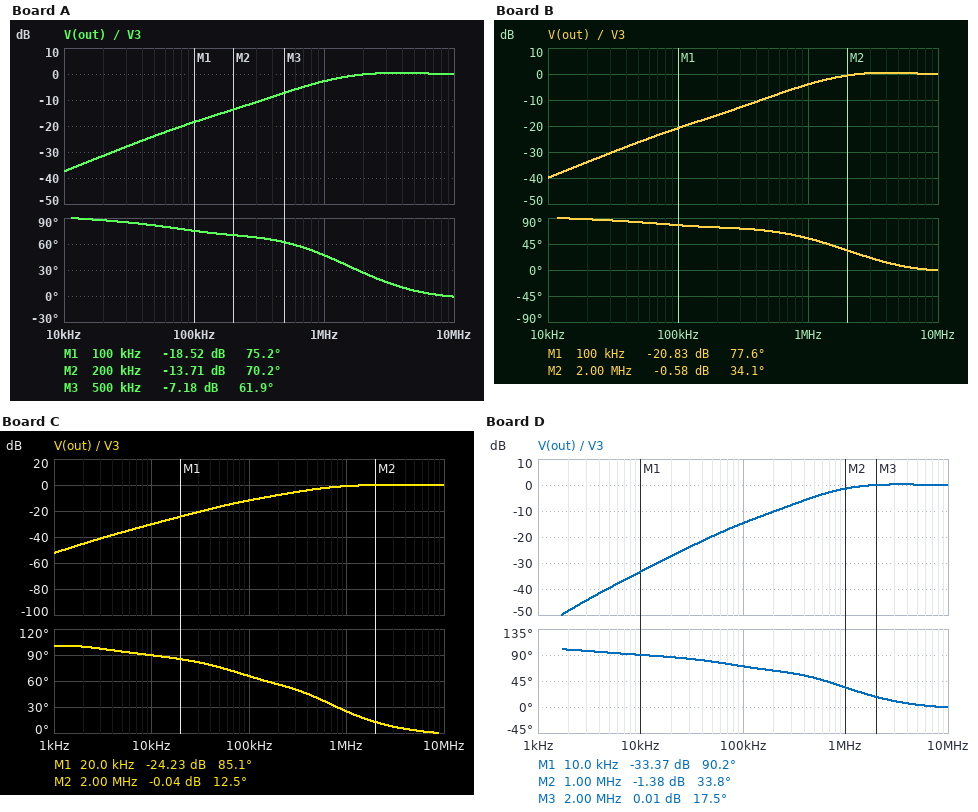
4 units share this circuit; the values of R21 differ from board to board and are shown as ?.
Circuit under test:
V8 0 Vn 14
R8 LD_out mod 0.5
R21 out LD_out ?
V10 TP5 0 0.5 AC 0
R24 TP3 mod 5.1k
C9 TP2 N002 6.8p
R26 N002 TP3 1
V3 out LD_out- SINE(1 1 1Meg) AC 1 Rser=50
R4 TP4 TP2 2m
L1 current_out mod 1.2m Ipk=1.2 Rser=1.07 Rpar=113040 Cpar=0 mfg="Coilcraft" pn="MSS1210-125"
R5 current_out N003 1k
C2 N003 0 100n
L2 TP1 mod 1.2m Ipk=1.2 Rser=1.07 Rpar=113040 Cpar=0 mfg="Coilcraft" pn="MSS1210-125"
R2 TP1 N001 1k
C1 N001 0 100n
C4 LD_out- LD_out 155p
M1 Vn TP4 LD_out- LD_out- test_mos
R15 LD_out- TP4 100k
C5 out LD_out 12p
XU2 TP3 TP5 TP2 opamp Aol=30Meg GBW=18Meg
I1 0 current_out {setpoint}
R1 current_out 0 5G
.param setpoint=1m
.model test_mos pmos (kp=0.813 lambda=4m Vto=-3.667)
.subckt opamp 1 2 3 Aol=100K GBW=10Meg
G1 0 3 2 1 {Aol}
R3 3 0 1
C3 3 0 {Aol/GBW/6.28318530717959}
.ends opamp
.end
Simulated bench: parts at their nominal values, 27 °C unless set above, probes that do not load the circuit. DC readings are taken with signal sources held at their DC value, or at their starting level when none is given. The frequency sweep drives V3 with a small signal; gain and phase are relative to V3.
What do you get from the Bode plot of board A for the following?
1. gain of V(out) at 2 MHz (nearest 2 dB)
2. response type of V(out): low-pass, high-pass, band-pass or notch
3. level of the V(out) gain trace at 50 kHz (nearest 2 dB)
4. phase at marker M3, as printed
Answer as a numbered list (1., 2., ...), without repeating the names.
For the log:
1. 0 dB
2. high-pass
3. -24 dB
4. 61.9 deg
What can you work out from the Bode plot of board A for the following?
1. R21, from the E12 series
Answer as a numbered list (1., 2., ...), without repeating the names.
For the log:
1. 680 Ω
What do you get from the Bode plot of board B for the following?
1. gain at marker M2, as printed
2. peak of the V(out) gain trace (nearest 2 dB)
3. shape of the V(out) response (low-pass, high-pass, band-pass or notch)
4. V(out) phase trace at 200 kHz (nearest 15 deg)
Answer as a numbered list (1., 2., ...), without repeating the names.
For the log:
1. -0.58 dB
2. 0 dB
3. high-pass
4. 75 deg
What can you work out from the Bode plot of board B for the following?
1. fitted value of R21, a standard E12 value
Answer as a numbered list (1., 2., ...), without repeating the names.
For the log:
1. 470 Ω
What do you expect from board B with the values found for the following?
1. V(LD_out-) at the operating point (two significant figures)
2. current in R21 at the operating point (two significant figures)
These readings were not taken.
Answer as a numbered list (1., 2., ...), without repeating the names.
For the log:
1. -1.0 V
2. 1.0 mA
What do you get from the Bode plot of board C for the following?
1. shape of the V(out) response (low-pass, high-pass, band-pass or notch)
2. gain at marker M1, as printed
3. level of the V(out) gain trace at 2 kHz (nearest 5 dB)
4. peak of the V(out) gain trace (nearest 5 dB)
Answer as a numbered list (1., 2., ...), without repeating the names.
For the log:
1. high-pass
2. -24.23 dB
3. -45 dB
4. 0 dB
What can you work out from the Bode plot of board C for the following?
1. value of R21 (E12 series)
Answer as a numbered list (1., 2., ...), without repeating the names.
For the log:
1. 1.8 kΩ
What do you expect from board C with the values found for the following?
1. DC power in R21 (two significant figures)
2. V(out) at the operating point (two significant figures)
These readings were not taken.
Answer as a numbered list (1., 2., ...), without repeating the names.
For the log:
1. 1.8 mW
2. -1.3 V
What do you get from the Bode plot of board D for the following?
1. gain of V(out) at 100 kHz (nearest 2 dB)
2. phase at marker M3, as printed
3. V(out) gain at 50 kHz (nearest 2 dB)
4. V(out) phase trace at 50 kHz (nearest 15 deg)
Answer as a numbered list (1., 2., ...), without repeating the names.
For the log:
1. -14 dB
2. 17.5 deg
3. -20 dB
4. 75 deg
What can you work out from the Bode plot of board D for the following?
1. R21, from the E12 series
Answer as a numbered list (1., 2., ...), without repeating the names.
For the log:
1. 1.2 kΩ
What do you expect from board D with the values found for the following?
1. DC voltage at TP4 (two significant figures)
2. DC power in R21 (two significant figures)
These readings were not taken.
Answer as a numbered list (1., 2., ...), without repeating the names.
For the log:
1. -5.5 V
2. 1.2 mW
